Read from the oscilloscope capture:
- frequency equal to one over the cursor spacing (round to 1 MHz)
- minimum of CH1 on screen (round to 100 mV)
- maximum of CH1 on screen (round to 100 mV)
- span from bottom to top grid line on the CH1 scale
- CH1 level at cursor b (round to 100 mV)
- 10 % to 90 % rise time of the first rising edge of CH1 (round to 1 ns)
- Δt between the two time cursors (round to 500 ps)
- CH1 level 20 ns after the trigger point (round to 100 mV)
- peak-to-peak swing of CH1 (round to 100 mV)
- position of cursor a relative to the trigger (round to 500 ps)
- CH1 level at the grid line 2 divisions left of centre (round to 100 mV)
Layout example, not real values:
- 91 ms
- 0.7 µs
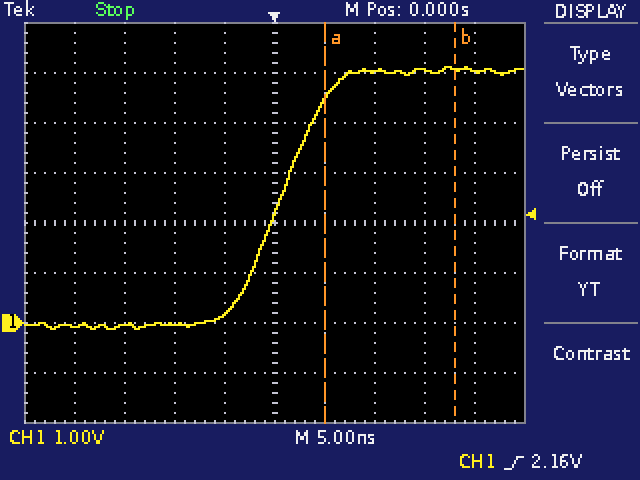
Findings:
- 77 MHz
- -100 mV
- 5.1 V
- 8 V
- 5.1 V
- 9 ns
- 13.0 ns
- 5.0 V
- 5.2 V
- +5.0 ns
- 0.0 V
